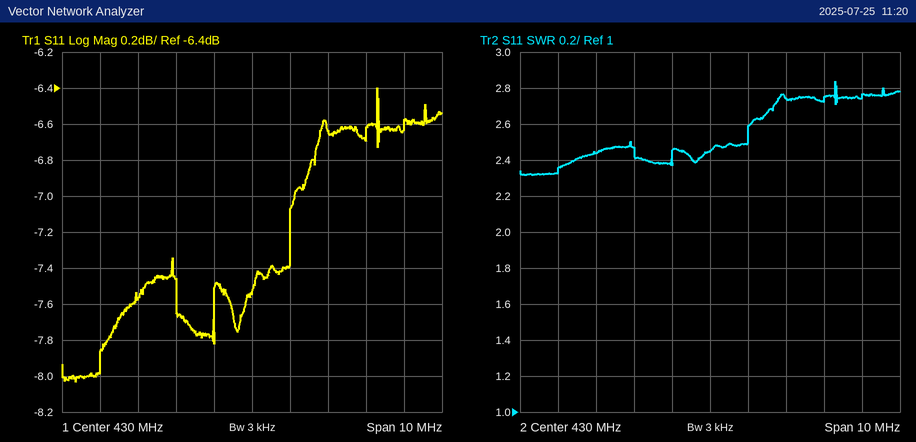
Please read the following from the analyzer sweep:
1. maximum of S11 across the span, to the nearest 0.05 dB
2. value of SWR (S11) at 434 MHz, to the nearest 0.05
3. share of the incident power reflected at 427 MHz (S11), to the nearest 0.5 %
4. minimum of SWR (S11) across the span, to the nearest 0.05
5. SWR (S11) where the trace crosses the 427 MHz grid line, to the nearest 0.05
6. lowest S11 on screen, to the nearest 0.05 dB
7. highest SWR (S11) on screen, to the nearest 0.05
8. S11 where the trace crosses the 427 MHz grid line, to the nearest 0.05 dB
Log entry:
-6.40 dB
2.75
17.5 %
2.30
2.45
-8.05 dB
2.85
-7.55 dB
